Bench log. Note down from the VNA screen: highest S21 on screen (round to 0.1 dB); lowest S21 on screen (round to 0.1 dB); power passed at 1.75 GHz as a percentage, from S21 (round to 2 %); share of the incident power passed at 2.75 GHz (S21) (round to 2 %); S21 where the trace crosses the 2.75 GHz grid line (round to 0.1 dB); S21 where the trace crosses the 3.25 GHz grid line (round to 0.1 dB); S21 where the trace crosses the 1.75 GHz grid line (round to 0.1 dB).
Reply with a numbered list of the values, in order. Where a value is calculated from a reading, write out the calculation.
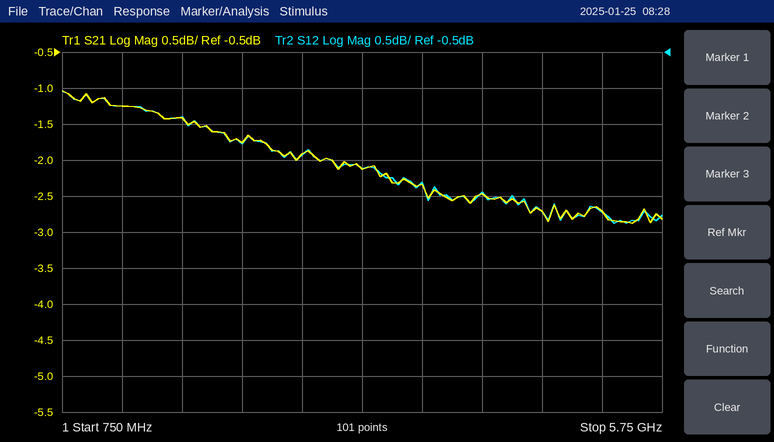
1. -1.0 dB
2. -2.9 dB
3. 10^(-1.4/10) ≈ 72 %
4. 10^(-1.9/10) ≈ 64.6 %, so 64 % to the nearest 2 %
5. -1.9 dB
6. -2.1 dB
7. -1.4 dB
